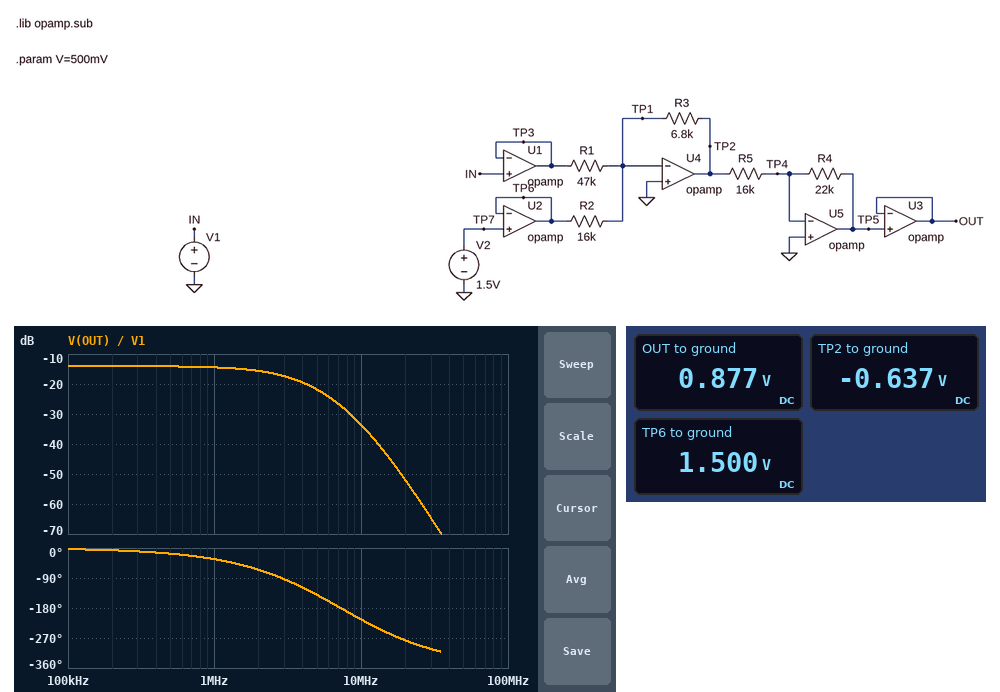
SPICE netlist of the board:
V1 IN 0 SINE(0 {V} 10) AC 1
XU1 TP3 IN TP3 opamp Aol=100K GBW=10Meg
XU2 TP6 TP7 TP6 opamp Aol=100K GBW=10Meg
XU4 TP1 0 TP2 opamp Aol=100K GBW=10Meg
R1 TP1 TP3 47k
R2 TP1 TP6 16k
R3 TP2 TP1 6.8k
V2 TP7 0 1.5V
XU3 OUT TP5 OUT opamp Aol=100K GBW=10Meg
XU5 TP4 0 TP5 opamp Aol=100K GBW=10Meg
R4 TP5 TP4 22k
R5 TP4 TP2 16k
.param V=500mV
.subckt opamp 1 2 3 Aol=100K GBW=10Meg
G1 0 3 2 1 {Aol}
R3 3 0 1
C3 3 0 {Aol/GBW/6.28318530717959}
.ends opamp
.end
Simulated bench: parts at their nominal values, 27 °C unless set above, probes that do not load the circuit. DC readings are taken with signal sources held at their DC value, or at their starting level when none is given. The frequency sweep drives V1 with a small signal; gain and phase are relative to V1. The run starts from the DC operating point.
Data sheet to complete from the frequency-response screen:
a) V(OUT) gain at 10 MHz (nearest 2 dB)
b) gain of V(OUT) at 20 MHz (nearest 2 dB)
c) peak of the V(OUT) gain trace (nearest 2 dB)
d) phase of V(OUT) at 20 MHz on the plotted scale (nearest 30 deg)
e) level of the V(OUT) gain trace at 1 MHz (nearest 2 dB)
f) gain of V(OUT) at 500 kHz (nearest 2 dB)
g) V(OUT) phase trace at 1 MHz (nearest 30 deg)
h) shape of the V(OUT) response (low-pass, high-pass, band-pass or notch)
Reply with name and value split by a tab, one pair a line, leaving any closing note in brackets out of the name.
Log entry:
V(OUT) gain at 10 MHz	-34 dB
gain of V(OUT) at 20 MHz	-52 dB
peak of the V(OUT) gain trace	-14 dB
phase of V(OUT) at 20 MHz on the plotted scale	-270 deg
level of the V(OUT) gain trace at 1 MHz	-14 dB
gain of V(OUT) at 500 kHz	-14 dB
V(OUT) phase trace at 1 MHz	-30 deg
shape of the V(OUT) response	low-pass
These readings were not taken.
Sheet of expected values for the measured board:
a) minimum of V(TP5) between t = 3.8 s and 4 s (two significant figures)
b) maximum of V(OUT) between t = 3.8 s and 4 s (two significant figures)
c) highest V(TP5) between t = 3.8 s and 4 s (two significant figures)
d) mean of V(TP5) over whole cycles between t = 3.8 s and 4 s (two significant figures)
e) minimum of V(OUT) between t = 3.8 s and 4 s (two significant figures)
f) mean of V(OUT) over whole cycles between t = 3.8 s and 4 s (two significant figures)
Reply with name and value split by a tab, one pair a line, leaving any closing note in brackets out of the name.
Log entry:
minimum of V(TP5) between t = 3.8 s and 4 s	780 mV
maximum of V(OUT) between t = 3.8 s and 4 s	980 mV
highest V(TP5) between t = 3.8 s and 4 s	980 mV
mean of V(TP5) over whole cycles between t = 3.8 s and 4 s	880 mV
minimum of V(OUT) between t = 3.8 s and 4 s	780 mV
mean of V(OUT) over whole cycles between t = 3.8 s and 4 s	880 mV
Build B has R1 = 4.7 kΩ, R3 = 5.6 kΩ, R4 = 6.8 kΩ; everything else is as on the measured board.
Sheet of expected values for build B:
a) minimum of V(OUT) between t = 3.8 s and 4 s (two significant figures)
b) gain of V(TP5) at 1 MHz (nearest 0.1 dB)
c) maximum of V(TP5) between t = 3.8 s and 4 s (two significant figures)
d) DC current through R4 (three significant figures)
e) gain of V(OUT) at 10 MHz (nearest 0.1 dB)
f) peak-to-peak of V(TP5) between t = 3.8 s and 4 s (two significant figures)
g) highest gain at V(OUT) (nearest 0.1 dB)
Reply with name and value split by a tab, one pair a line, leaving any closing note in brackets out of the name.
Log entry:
minimum of V(OUT) between t = 3.8 s and 4 s	-30 mV
gain of V(TP5) at 1 MHz	-6.3 dB
maximum of V(TP5) between t = 3.8 s and 4 s	480 mV
DC current through R4	32.8 µA
gain of V(OUT) at 10 MHz	-25.5 dB
peak-to-peak of V(TP5) between t = 3.8 s and 4 s	510 mV
highest gain at V(OUT)	-5.9 dB
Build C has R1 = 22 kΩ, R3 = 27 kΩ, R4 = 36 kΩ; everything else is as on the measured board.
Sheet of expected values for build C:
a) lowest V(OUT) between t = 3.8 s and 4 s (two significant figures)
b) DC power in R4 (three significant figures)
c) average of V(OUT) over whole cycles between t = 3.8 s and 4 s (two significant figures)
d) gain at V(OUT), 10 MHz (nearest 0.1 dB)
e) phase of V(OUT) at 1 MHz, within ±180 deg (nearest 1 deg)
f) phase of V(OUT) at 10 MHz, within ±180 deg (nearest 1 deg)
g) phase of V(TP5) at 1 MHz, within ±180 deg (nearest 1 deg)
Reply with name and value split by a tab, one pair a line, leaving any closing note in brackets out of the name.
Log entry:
lowest V(OUT) between t = 3.8 s and 4 s	4.3 V
DC power in R4	901 µW
average of V(OUT) over whole cycles between t = 3.8 s and 4 s	5.7 V
gain at V(OUT), 10 MHz	-20.0 dB
phase of V(OUT) at 1 MHz, within ±180 deg	-51 deg
phase of V(OUT) at 10 MHz, within ±180 deg	121 deg
phase of V(TP5) at 1 MHz, within ±180 deg	-45 deg
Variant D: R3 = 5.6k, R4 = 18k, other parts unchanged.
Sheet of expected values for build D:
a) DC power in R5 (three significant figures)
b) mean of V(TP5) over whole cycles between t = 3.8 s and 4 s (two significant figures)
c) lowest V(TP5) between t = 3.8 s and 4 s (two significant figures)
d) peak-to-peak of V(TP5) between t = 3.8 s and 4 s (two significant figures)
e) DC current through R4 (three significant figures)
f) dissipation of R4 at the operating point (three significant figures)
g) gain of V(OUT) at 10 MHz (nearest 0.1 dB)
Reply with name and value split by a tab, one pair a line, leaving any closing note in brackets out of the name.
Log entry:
DC power in R5	17.2 µW
mean of V(TP5) over whole cycles between t = 3.8 s and 4 s	590 mV
lowest V(TP5) between t = 3.8 s and 4 s	520 mV
peak-to-peak of V(TP5) between t = 3.8 s and 4 s	130 mV
DC current through R4	32.8 µA
dissipation of R4 at the operating point	19.4 µW
gain of V(OUT) at 10 MHz	-35.9 dB
